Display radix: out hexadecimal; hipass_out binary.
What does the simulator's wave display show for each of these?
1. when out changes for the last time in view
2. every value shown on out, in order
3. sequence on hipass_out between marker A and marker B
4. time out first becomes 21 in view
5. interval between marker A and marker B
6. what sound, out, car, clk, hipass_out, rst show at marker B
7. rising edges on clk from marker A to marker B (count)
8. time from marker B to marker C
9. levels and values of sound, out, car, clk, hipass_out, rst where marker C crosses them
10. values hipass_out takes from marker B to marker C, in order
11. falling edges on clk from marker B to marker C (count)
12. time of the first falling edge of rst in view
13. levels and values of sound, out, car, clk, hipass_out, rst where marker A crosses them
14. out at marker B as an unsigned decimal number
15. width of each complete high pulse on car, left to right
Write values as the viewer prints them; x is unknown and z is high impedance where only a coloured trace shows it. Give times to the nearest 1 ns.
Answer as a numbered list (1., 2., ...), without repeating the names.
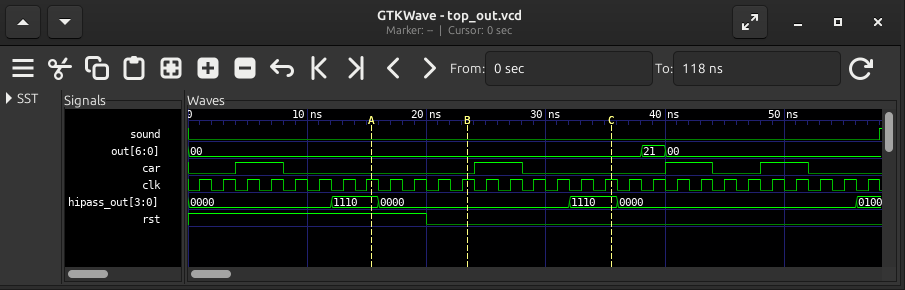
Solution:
1. 40 ns
2. 00, 21, 00
3. 1110, 0000
4. 38 ns
5. 8 ns
6. sound=0, out=00, car=0, clk=1, hipass_out=0000, rst=0
7. 4
8. 12 ns
9. sound=0, out=00, car=0, clk=1, hipass_out=1110, rst=0
10. 0000, 1110
11. 6
12. 20 ns
13. sound=0, out=00, car=0, clk=1, hipass_out=1110, rst=1
14. 0
15. 4 ns, 4 ns, 4 ns, 4 ns
